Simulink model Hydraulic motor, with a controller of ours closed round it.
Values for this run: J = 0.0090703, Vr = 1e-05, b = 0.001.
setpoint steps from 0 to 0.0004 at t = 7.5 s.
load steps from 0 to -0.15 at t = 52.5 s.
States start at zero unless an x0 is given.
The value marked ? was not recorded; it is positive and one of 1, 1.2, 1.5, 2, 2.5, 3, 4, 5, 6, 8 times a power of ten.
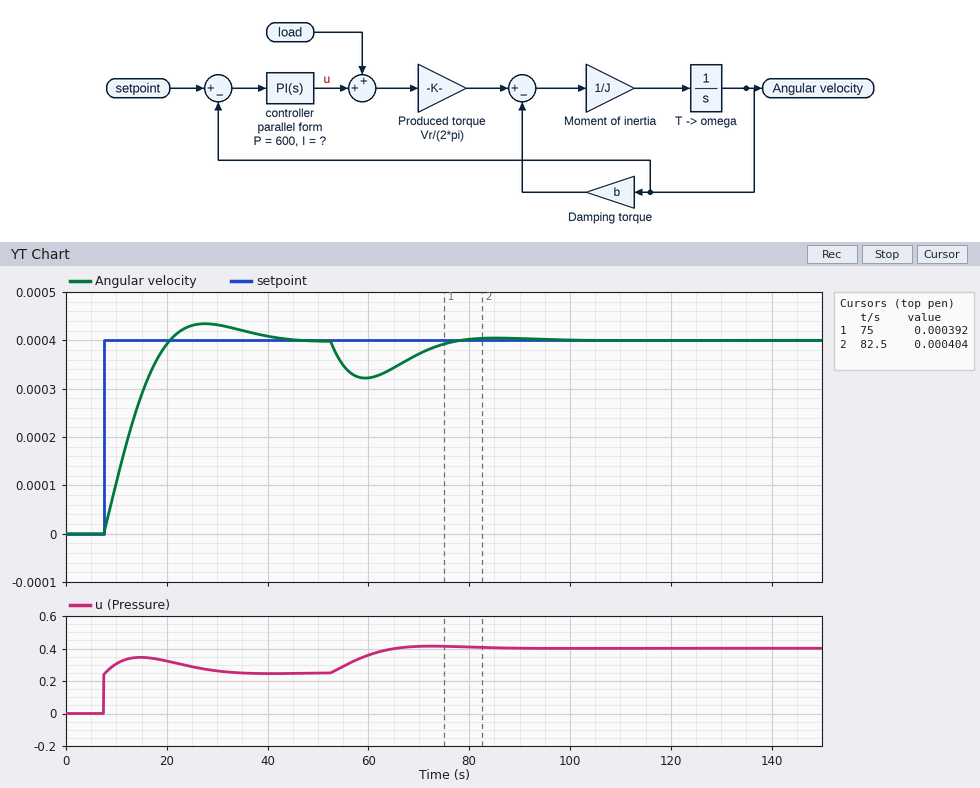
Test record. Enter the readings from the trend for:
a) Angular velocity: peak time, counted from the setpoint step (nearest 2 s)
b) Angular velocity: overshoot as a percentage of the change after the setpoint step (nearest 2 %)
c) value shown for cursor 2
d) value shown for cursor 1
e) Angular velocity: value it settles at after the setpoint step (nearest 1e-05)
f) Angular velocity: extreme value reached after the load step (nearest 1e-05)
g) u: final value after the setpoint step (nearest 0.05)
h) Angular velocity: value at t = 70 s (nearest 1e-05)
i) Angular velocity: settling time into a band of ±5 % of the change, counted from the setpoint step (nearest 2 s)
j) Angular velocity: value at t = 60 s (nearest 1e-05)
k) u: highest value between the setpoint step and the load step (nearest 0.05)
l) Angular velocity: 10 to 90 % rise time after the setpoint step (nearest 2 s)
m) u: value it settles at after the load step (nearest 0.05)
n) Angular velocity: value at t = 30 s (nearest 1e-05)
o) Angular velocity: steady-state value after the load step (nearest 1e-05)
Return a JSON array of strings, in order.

["20 s", "8 %", "0.000404", "0.000392", "0.00040", "0.00032", "0.25", "0.00037", "28 s", "0.00032", "0.35", "10 s", "0.40", "0.00043", "0.00040"]
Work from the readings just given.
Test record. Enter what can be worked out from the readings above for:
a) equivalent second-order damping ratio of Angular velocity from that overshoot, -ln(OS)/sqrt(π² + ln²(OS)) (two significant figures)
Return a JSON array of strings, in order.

["0.63"]
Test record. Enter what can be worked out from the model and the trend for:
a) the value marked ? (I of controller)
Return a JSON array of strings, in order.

["150"]
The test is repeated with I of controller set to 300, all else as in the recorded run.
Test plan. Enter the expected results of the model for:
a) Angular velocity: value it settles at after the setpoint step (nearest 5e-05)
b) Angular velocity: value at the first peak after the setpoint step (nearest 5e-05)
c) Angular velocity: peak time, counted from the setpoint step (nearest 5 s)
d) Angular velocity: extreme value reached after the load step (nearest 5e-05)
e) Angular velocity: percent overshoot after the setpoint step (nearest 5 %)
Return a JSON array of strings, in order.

["0.00040", "0.00050", "15 s", "0.00035", "20 %"]
